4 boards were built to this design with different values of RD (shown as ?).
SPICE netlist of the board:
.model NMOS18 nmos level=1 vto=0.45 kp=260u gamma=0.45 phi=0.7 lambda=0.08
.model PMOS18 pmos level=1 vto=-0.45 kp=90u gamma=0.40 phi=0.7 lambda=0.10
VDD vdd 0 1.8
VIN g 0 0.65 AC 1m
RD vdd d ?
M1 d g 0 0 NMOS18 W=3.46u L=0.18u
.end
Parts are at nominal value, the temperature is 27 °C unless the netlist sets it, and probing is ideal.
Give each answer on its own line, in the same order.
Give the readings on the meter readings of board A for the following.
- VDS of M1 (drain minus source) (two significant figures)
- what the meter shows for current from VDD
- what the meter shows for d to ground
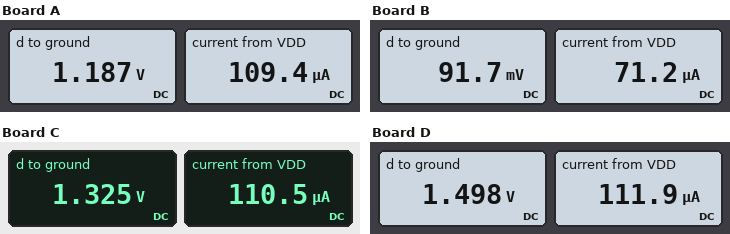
1.2 V
109.4 µA
1.187 V
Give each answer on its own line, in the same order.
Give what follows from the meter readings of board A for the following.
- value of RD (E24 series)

5.6 kΩ
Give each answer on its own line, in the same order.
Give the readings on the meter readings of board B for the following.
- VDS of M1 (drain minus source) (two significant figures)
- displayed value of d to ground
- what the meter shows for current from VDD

92 mV
91.7 mV
71.2 µA
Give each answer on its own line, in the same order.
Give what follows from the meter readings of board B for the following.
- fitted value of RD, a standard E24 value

24 kΩ
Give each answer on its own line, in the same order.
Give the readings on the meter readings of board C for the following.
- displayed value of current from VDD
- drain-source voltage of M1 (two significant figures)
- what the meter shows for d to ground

110.5 µA
1.3 V
1.325 V
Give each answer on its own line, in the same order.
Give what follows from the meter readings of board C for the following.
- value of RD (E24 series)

4.3 kΩ
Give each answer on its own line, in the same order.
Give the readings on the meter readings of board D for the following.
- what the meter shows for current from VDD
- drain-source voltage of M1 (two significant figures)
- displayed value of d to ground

111.9 µA
1.5 V
1.498 V
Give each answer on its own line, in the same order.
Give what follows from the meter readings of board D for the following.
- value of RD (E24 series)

2.7 kΩ
